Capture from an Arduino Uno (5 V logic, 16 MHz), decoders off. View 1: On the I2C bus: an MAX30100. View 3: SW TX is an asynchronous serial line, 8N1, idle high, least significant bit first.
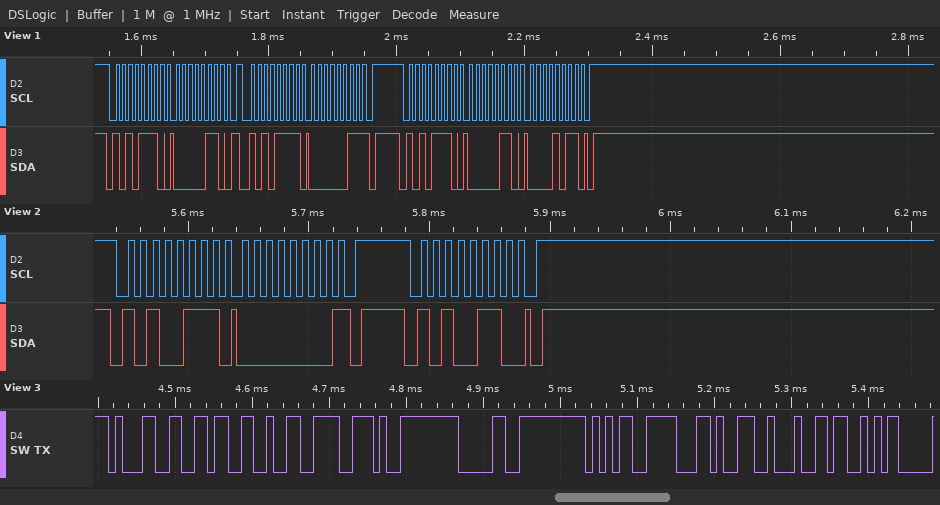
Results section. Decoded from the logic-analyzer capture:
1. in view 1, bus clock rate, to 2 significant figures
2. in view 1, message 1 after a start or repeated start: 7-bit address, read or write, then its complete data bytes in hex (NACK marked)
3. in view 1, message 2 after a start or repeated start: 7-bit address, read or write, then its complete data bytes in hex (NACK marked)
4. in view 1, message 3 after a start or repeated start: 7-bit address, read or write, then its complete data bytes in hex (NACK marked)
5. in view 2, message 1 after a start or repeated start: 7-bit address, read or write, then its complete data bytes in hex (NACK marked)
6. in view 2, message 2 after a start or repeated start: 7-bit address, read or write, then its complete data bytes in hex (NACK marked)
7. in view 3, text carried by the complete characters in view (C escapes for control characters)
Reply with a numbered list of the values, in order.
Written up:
1. 100 kHz
2. 0x57 write: 06
3. 0x57 read: 03 NACK
4. 0x57 write: 06 0B
5. 0x53 read: 00 NACK
6. 0x53 write
7. "162.05,\"S"
